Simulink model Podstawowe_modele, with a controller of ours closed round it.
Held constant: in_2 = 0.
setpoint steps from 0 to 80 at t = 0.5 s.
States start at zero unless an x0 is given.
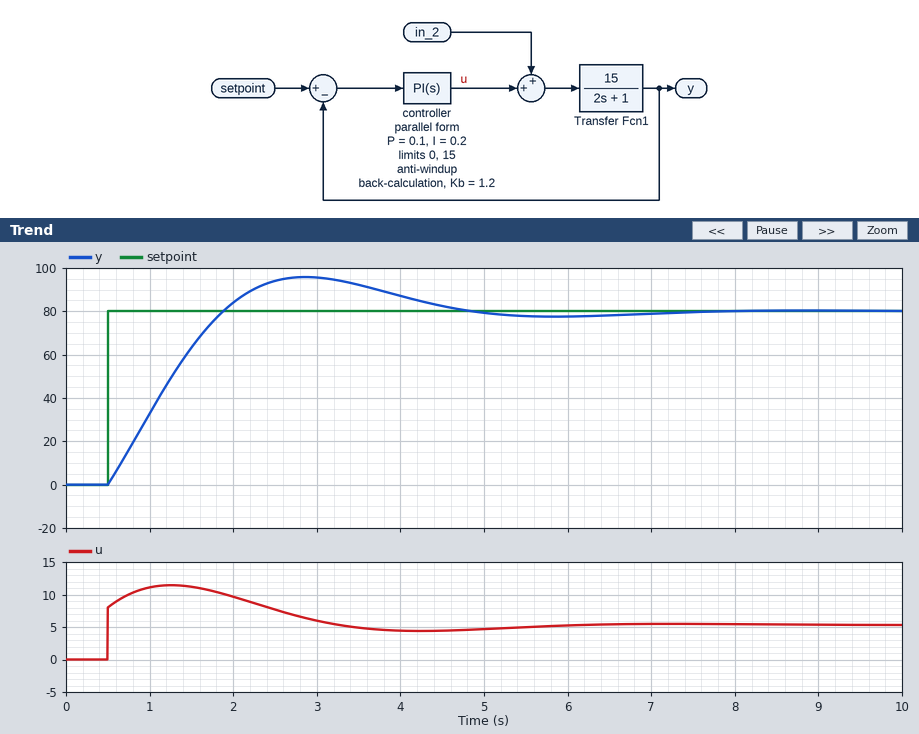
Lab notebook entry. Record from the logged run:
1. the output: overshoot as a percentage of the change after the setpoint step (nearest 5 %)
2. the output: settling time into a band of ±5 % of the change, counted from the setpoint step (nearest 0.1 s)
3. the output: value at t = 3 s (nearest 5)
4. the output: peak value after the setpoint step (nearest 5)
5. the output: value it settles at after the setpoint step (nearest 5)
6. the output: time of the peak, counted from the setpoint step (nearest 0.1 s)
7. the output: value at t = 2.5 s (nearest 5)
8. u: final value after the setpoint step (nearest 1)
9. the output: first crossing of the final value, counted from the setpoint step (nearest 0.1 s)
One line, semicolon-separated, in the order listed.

20 %; 3.8 s; 95; 95; 80; 2.4 s; 95; 5; 1.4 s
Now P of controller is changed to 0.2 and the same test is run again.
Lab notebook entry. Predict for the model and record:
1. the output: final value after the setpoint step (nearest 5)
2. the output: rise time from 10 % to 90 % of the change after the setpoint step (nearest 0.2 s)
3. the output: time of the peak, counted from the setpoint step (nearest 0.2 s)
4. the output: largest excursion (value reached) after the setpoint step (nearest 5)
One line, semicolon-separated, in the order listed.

80; 1.0 s; 2.2 s; 85
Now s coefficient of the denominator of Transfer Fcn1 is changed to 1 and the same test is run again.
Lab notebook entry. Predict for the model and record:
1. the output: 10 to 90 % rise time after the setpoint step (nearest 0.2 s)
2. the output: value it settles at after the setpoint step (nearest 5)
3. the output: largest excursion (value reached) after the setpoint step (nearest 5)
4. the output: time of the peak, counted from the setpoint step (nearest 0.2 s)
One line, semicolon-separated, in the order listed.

0.8 s; 80; 85; 1.8 s
